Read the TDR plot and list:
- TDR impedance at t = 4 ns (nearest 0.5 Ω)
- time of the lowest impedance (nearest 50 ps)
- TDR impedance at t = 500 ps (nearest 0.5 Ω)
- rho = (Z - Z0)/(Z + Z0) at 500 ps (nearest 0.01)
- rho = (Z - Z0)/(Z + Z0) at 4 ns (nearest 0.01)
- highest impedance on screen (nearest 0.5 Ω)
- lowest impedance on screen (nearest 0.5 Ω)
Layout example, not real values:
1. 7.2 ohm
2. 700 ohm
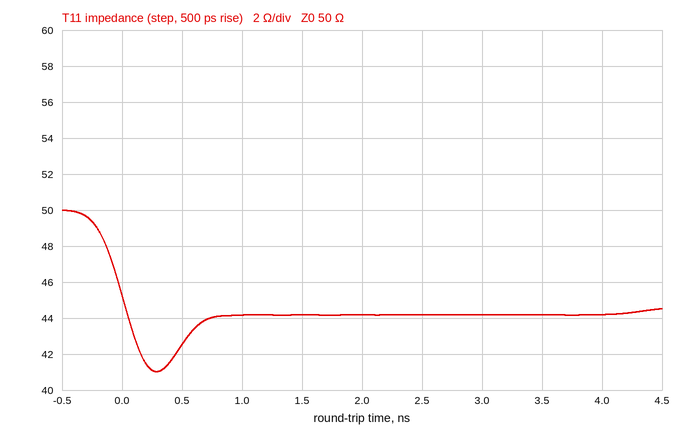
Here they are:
1. 44.0 Ω
2. 300 ps
3. 42.5 Ω
4. -0.08
5. -0.06
6. 50.0 Ω
7. 41.0 Ω
